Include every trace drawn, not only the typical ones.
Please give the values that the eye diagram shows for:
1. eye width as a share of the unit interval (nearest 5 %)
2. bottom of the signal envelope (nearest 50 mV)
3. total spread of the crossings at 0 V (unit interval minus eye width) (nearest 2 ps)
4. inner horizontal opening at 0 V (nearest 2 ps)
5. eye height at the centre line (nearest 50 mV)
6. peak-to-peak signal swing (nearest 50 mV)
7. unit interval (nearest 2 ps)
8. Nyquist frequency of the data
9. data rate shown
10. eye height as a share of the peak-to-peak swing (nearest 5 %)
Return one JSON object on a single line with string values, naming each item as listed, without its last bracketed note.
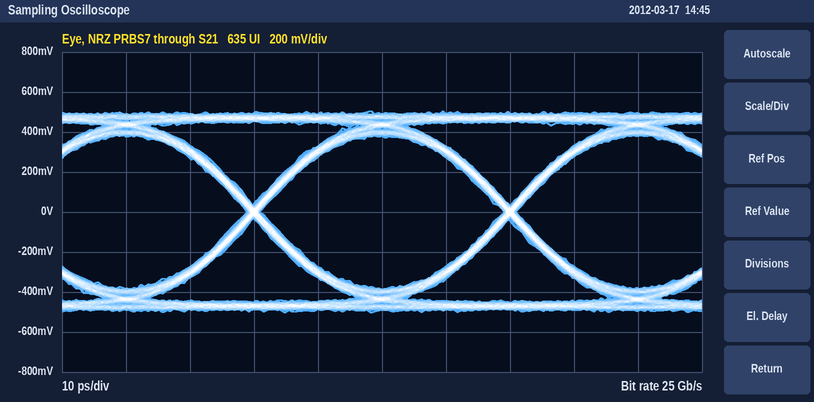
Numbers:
{"eye width as a share of the unit interval": "95 %", "bottom of the signal envelope": "-500 mV", "total spread of the crossings at 0 V (unit interval minus eye width)": "2 ps", "inner horizontal opening at 0 V": "38 ps", "eye height at the centre line": "750 mV", "peak-to-peak signal swing": "1.00 V", "unit interval": "40 ps", "Nyquist frequency of the data": "12.5 GHz", "data rate shown": "25 Gb/s", "eye height as a share of the peak-to-peak swing": "75 %"}
